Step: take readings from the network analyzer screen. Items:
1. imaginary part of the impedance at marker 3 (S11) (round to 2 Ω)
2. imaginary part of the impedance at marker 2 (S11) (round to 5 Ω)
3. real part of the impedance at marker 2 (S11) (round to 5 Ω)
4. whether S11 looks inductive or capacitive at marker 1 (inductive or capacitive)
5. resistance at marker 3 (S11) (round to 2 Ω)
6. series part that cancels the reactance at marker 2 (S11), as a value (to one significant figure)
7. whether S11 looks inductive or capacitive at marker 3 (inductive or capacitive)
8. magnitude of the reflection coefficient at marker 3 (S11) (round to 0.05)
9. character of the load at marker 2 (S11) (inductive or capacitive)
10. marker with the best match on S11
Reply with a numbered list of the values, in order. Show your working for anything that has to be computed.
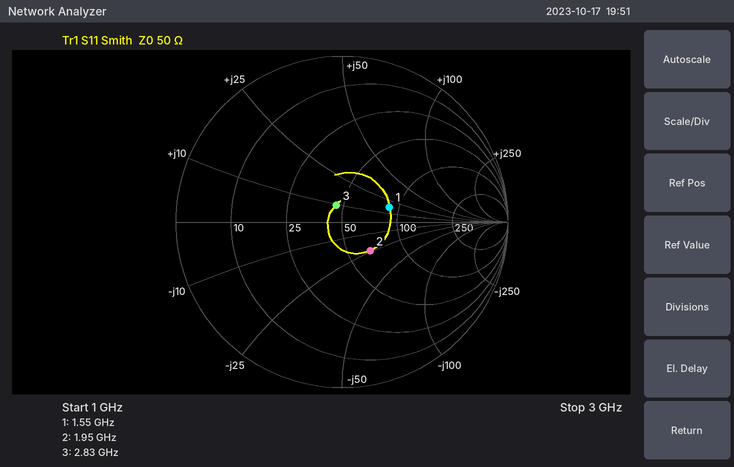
1. +10 Ω
2. -25 Ω
3. 65 Ω
4. inductive
5. 46 Ω
6. L = 25 Ω/(2π × 1.95 GHz) ≈ 2 nH
7. inductive
8. 0.10
9. capacitive
10. marker 3
